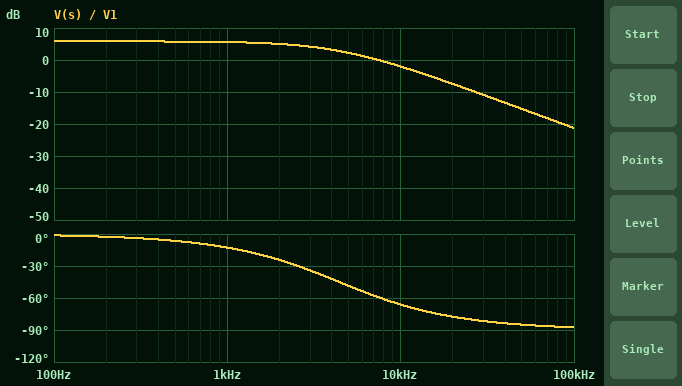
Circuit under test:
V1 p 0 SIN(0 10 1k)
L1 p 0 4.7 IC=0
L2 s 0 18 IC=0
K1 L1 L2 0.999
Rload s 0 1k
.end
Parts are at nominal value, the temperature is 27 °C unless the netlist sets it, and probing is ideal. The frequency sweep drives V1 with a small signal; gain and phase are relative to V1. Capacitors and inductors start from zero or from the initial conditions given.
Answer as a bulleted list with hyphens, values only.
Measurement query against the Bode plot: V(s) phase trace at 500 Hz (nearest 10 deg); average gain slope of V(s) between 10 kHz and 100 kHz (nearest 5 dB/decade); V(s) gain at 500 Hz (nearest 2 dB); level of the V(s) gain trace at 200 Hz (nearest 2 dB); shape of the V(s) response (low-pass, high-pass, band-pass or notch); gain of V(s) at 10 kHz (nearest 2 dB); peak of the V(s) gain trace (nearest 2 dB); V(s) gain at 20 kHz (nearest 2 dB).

- -10 deg
- -20 dB/decade
- 6 dB
- 6 dB
- low-pass
- -2 dB
- 6 dB
- -8 dB
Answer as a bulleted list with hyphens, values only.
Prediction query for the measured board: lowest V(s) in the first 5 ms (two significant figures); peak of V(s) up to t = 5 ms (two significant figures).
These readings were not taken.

- -19 V
- 19 V
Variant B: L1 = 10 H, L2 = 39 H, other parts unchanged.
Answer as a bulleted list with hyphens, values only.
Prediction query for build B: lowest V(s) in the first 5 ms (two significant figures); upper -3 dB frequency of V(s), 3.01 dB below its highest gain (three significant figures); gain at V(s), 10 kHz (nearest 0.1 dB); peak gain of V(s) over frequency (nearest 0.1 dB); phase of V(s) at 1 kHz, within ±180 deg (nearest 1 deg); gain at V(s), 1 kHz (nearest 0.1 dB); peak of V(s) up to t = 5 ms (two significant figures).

- -18 V
- 2.04 kHz
- -8.1 dB
- 5.9 dB
- -26 deg
- 5.0 dB
- 18 V
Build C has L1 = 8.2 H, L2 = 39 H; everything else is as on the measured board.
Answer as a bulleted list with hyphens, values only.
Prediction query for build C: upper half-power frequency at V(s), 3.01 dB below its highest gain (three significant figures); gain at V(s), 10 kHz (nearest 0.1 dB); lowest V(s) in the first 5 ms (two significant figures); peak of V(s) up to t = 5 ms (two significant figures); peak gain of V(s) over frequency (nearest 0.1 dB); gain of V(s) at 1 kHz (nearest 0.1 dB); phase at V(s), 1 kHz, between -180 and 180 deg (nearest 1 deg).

- 2.04 kHz
- -7.2 dB
- -20 V
- 20 V
- 6.8 dB
- 5.8 dB
- -26 deg
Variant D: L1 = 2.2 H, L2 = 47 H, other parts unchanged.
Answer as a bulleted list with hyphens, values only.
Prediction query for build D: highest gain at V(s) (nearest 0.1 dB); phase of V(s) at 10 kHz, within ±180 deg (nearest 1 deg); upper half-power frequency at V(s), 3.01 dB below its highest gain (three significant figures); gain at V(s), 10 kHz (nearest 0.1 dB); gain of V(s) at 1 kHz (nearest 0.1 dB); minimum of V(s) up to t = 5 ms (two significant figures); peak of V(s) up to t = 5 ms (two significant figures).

- 13.3 dB
- -80 deg
- 1.69 kHz
- -2.3 dB
- 12.0 dB
- -40 V
- 40 V
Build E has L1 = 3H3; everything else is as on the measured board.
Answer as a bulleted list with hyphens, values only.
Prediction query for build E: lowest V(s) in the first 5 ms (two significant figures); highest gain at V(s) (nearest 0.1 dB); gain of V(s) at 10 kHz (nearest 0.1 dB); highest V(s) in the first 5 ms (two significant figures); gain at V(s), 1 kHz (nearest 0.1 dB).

- -23 V
- 7.4 dB
- -0.5 dB
- 23 V
- 7.1 dB
